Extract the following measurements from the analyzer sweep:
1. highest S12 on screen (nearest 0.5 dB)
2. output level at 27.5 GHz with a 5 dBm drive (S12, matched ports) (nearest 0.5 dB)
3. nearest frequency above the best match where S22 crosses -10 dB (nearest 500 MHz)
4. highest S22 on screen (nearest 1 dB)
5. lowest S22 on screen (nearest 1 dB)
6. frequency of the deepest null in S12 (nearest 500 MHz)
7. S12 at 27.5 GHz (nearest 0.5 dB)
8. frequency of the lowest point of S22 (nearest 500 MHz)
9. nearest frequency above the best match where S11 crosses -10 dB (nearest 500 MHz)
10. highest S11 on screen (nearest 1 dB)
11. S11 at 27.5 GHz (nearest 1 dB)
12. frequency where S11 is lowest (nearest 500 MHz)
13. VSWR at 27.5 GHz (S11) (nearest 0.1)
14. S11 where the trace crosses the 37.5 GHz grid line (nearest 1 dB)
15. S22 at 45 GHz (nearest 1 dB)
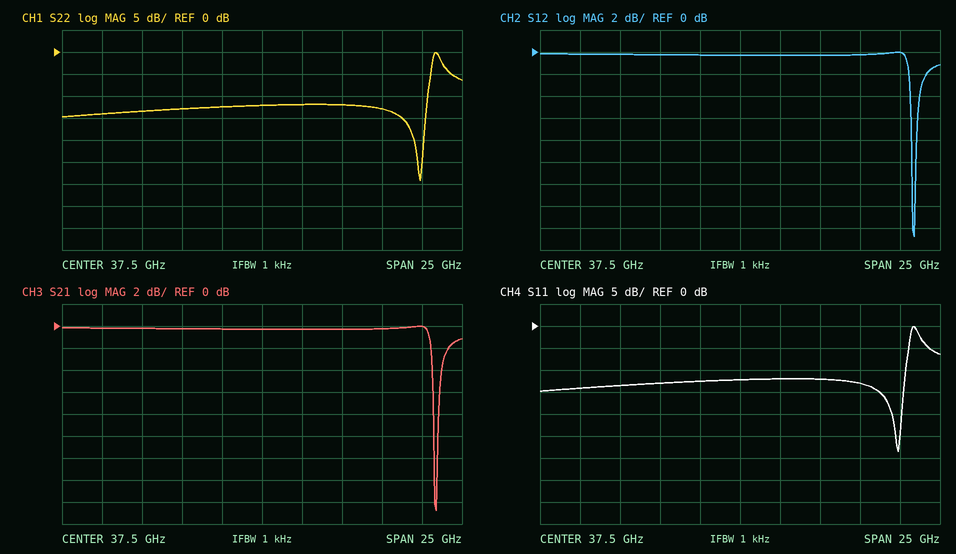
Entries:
0.0 dB
5.0 dBm
48.0 GHz
0 dB
-29 dB
48.5 GHz
0.0 dB
47.5 GHz
48.0 GHz
0 dB
-14 dB
47.5 GHz
1.5
-12 dB
-13 dB
